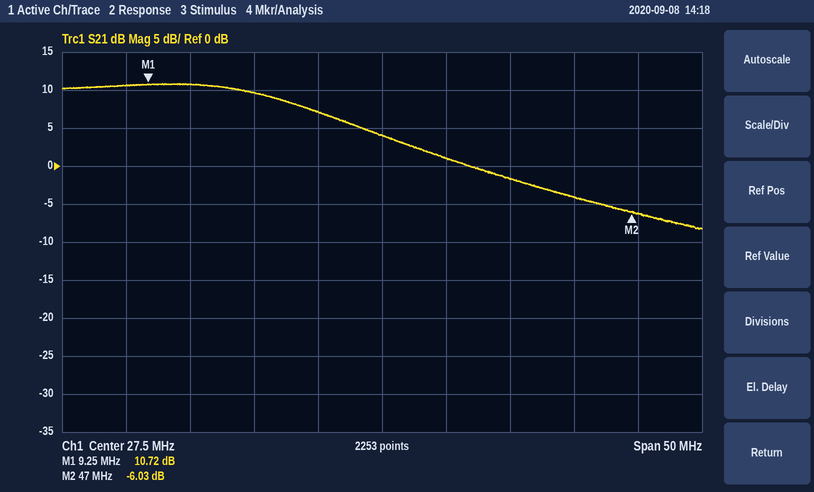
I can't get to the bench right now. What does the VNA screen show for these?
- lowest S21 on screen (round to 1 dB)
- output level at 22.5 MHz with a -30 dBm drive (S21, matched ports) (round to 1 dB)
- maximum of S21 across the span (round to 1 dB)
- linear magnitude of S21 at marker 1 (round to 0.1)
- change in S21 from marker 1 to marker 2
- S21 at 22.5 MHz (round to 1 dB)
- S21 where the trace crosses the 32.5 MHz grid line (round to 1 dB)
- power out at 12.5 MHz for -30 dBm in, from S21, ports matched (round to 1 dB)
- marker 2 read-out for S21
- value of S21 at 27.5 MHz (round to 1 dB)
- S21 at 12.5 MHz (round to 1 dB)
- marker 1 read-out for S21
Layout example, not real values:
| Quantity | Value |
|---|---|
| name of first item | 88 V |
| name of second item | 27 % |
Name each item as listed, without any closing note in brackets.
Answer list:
| Quantity | Value |
|---|---|
| lowest S21 on screen | -8 dB |
| output level at 22.5 MHz with a -30 dBm drive (S21, matched ports) | -23 dBm |
| maximum of S21 across the span | 11 dB |
| linear magnitude of S21 at marker 1 | 3.4 |
| change in S21 from marker 1 to marker 2 | -16.75 dB |
| S21 at 22.5 MHz | 7 dB |
| S21 where the trace crosses the 32.5 MHz grid line | 1 dB |
| power out at 12.5 MHz for -30 dBm in, from S21, ports matched | -19 dBm |
| marker 2 read-out for S21 | -6.03 dB |
| value of S21 at 27.5 MHz | 4 dB |
| S21 at 12.5 MHz | 11 dB |
| marker 1 read-out for S21 | 10.72 dB |
